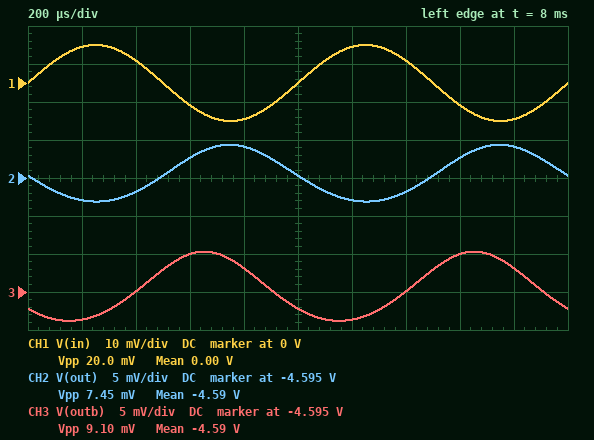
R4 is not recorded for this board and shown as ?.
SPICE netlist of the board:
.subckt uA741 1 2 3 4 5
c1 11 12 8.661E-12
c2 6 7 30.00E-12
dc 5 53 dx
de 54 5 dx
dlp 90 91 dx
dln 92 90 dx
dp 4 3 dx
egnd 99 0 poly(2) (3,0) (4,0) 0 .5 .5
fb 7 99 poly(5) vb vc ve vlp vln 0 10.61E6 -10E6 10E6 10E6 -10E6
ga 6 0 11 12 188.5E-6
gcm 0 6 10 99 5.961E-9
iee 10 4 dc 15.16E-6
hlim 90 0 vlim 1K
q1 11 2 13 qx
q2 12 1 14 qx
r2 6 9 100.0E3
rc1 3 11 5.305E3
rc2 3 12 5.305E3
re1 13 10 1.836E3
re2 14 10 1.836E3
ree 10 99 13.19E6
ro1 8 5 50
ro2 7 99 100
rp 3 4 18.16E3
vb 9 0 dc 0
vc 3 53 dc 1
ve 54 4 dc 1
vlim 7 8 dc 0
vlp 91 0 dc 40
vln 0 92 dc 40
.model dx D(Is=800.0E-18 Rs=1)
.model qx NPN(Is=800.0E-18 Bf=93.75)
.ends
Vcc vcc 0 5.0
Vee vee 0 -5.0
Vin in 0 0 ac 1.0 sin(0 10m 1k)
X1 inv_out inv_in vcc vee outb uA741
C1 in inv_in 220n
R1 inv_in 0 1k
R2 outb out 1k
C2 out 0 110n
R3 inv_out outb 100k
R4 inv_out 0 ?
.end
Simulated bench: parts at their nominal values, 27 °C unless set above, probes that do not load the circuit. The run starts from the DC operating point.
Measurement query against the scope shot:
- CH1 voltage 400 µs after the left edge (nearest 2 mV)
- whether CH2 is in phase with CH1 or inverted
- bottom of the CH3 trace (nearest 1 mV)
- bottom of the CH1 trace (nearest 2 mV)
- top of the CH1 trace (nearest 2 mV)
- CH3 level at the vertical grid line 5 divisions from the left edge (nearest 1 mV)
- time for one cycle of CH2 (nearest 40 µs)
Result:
6 mV
inverted
-4.599 V
-10 mV
10 mV
-4.597 V
1.00 ms
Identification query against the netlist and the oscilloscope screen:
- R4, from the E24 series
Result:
910 Ω
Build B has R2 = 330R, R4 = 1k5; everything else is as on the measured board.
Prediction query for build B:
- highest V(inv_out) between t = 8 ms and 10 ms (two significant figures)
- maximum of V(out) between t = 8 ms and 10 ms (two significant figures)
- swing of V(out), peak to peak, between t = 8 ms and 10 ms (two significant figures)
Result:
-68 mV
-4.6 V
4.1 mV
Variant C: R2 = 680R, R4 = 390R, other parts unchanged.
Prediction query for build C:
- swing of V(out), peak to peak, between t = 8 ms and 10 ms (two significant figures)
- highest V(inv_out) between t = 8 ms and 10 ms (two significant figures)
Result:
23 mV
-18 mV
